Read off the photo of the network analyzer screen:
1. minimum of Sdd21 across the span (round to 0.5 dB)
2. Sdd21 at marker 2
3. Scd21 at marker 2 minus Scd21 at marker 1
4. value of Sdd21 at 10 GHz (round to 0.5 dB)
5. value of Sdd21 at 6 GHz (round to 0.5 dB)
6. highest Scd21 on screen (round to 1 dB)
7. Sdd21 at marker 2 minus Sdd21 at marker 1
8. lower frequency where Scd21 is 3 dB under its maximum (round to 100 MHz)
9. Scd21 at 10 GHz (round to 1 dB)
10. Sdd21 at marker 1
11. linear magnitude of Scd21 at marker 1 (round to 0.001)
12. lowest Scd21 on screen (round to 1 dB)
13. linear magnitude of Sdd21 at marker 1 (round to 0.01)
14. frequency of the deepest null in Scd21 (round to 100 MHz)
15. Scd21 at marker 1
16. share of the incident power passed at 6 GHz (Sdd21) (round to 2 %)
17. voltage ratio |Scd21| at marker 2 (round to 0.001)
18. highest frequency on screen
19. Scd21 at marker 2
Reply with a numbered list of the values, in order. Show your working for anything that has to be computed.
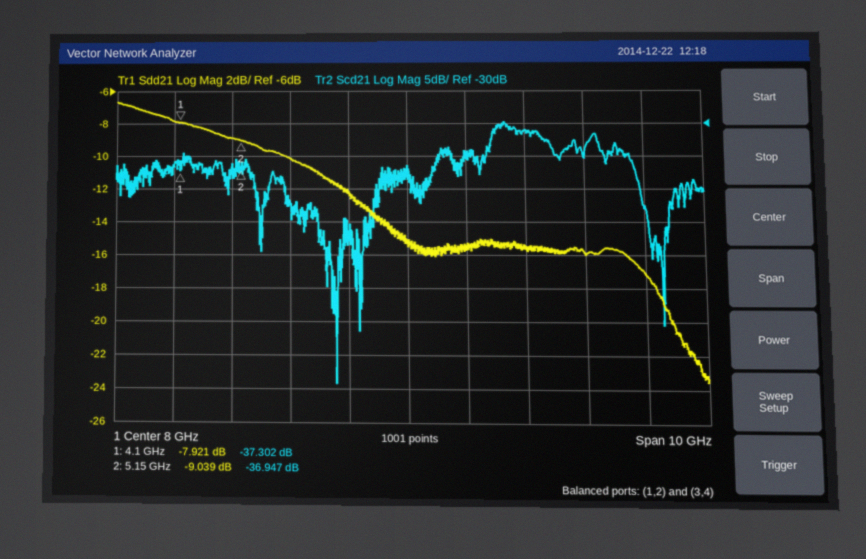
1. -23.5 dB
2. -9.039 dB
3. -36.947 − (-37.302) = 0.355 dB
4. -15.5 dB
5. -10.0 dB
6. -30 dB
7. -9.039 − (-7.921) = -1.118 dB
8. 9.4 GHz
9. -31 dB
10. -7.921 dB
11. 10^(-37.302/20) ≈ 0.014
12. -69 dB
13. 10^(-7.921/20) ≈ 0.40
14. 6.8 GHz
15. -37.302 dB
16. 10^(-10/10) ≈ 10 %
17. 10^(-36.947/20) ≈ 0.014
18. 13 GHz
19. -36.947 dB
